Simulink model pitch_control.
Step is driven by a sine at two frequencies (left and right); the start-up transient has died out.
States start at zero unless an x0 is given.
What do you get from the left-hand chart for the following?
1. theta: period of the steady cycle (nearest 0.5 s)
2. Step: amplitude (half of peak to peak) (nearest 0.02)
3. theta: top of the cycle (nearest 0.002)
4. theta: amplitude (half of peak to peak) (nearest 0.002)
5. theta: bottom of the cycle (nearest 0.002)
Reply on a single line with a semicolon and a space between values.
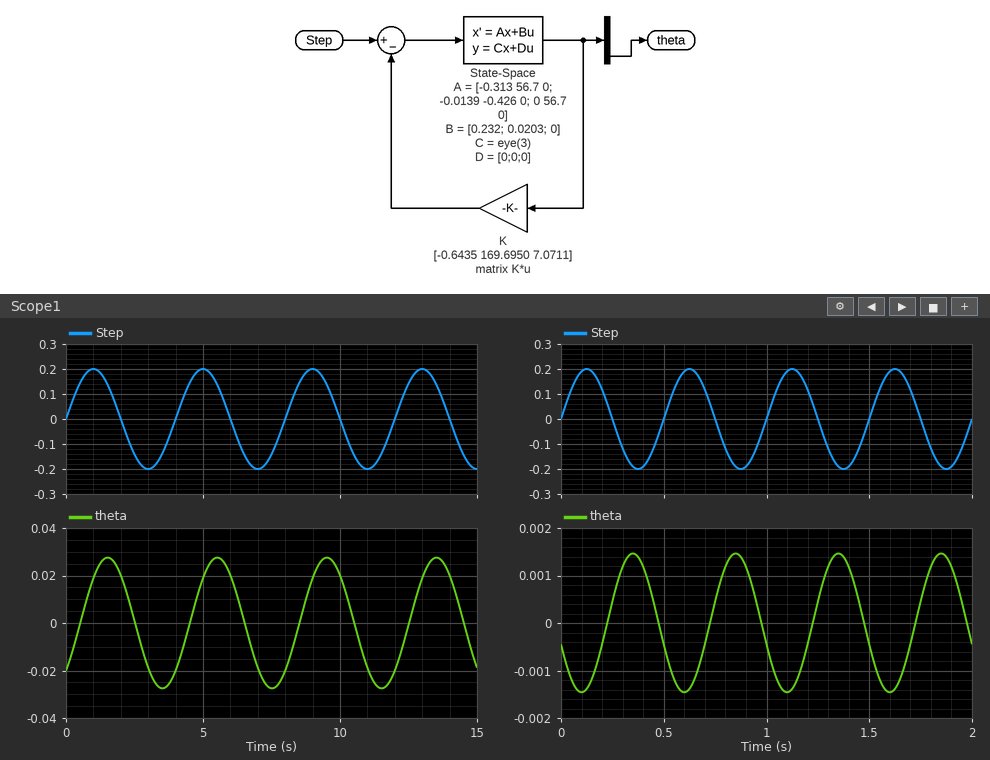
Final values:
4.0 s; 0.20; 0.028; 0.028; -0.028
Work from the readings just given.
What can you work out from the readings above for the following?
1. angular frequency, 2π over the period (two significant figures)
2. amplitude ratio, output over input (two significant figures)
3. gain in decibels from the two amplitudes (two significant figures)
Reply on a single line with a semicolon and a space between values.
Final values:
1.6 rad/s; 0.14; -17 dB
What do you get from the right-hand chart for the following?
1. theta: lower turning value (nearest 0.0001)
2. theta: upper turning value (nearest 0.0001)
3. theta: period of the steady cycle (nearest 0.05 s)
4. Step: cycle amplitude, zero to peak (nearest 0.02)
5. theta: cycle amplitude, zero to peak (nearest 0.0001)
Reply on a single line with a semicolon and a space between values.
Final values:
-0.0015; 0.0015; 0.50 s; 0.20; 0.0015
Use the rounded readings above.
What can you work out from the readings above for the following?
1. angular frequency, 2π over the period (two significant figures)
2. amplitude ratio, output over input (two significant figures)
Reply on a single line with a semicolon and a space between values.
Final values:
13 rad/s; 0.0075
